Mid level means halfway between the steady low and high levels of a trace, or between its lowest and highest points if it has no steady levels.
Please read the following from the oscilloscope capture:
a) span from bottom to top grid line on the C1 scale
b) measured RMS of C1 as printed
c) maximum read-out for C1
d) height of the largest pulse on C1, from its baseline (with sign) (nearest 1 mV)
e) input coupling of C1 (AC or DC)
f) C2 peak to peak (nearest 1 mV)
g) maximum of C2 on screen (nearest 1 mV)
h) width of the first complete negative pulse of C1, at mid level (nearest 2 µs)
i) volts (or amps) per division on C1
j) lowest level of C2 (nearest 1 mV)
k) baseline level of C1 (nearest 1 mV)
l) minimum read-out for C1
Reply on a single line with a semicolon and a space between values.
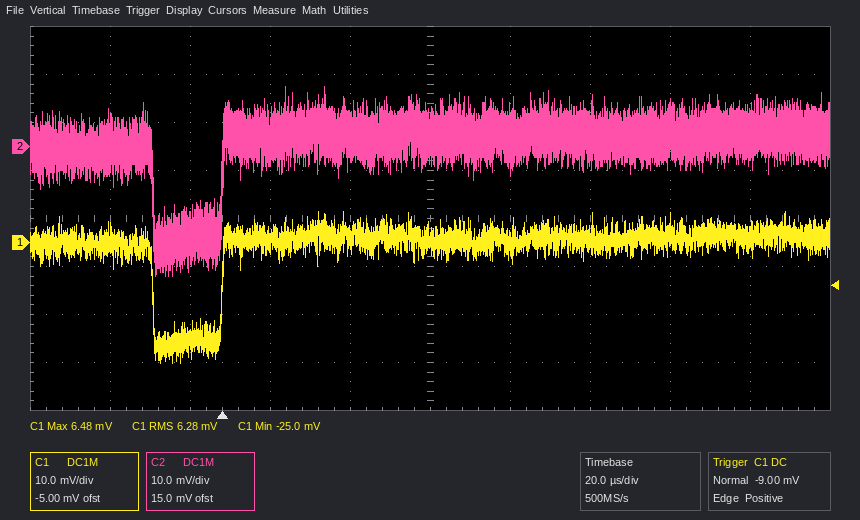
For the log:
80 mV; 6.28 mV; 6.48 mV; -26 mV; DC; 39 mV; 12 mV; 18 µs; 10 mV; -27 mV; 1 mV; -25.0 mV
